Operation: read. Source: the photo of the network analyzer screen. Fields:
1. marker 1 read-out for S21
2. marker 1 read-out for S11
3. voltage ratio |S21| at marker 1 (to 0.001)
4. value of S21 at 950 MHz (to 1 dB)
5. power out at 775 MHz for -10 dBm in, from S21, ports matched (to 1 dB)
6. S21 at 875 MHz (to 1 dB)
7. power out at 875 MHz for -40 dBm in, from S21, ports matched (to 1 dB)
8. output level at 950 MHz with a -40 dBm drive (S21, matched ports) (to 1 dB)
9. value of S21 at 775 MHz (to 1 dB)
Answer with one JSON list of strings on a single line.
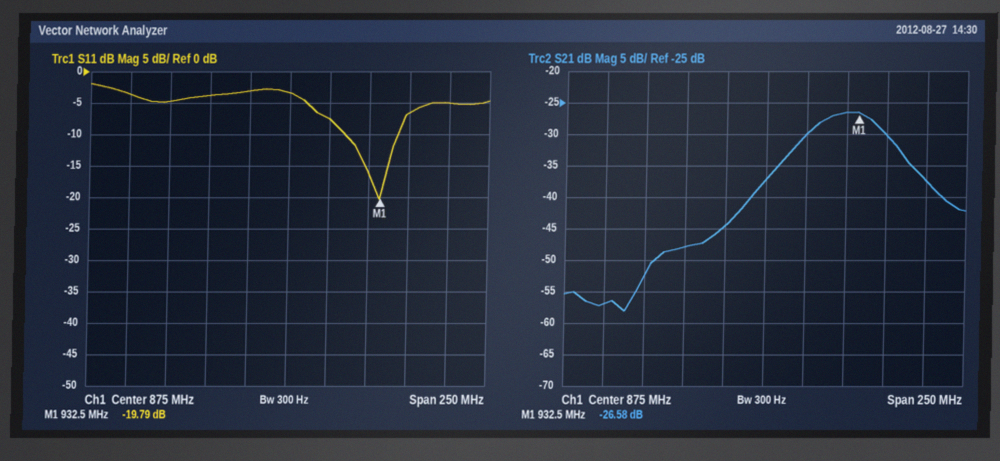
["-26.58 dB", "-19.79 dB", "0.047", "-30 dB", "-67 dBm", "-37 dB", "-77 dBm", "-70 dBm", "-57 dB"]
